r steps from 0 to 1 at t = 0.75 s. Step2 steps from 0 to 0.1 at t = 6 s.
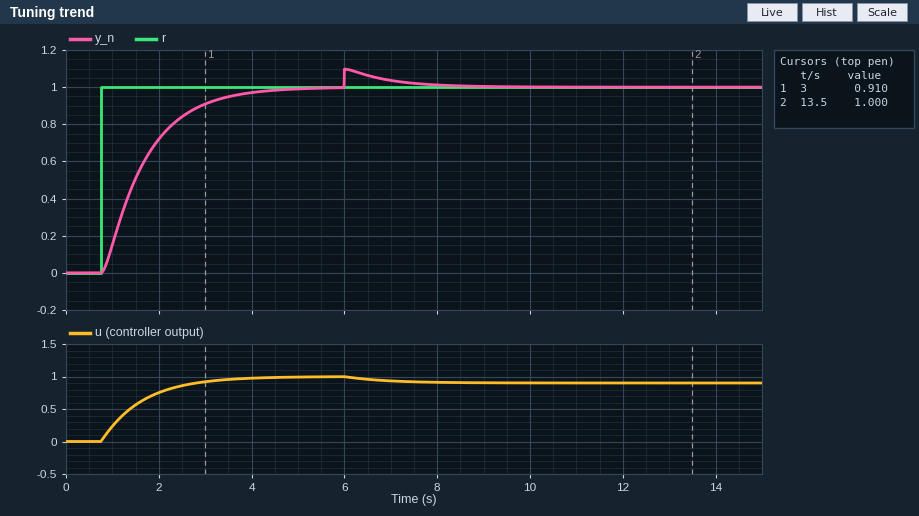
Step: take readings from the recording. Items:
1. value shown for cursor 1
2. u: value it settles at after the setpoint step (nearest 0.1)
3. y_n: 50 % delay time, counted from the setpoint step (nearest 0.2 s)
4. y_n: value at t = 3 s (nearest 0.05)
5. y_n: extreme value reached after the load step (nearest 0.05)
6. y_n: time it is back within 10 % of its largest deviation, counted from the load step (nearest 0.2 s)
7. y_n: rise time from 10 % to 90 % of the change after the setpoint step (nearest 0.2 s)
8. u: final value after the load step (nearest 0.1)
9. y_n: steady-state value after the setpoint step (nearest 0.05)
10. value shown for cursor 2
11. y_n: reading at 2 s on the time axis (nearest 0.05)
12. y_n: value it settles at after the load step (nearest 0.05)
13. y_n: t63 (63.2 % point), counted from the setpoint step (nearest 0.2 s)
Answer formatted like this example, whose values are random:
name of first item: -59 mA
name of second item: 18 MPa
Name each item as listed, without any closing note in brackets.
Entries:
value shown for cursor 1: 0.910
u: value it settles at after the setpoint step: 1.0
y_n: 50 % delay time, counted from the setpoint step: 0.8 s
y_n: value at t = 3 s: 0.90
y_n: extreme value reached after the load step: 1.10
y_n: time it is back within 10 % of its largest deviation, counted from the load step: 2.2 s
y_n: rise time from 10 % to 90 % of the change after the setpoint step: 2.0 s
u: final value after the load step: 0.9
y_n: steady-state value after the setpoint step: 1.00
value shown for cursor 2: 1.000
y_n: reading at 2 s on the time axis: 0.70
y_n: value it settles at after the load step: 1.00
y_n: t63 (63.2 % point), counted from the setpoint step: 1.0 s
